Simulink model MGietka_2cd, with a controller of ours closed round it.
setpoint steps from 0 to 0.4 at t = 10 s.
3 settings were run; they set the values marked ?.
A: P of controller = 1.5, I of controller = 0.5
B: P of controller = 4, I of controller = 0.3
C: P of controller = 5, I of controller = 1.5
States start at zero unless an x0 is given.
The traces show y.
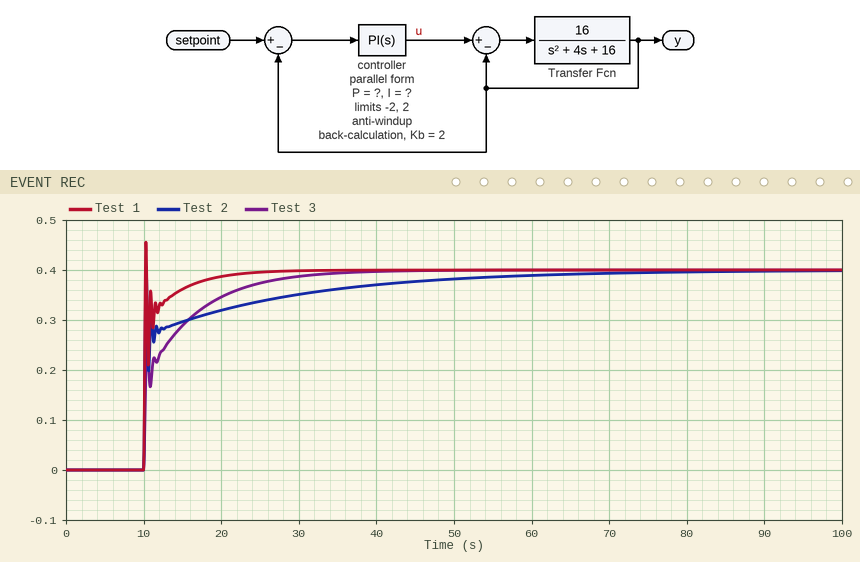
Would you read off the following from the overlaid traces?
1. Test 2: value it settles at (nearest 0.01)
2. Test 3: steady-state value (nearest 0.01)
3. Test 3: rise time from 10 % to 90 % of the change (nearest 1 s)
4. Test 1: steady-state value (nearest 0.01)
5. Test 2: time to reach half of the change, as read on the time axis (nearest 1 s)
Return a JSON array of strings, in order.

["0.40", "0.40", "12 s", "0.40", "10 s"]
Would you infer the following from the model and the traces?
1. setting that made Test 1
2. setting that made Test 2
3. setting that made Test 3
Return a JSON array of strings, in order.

["C", "B", "A"]
